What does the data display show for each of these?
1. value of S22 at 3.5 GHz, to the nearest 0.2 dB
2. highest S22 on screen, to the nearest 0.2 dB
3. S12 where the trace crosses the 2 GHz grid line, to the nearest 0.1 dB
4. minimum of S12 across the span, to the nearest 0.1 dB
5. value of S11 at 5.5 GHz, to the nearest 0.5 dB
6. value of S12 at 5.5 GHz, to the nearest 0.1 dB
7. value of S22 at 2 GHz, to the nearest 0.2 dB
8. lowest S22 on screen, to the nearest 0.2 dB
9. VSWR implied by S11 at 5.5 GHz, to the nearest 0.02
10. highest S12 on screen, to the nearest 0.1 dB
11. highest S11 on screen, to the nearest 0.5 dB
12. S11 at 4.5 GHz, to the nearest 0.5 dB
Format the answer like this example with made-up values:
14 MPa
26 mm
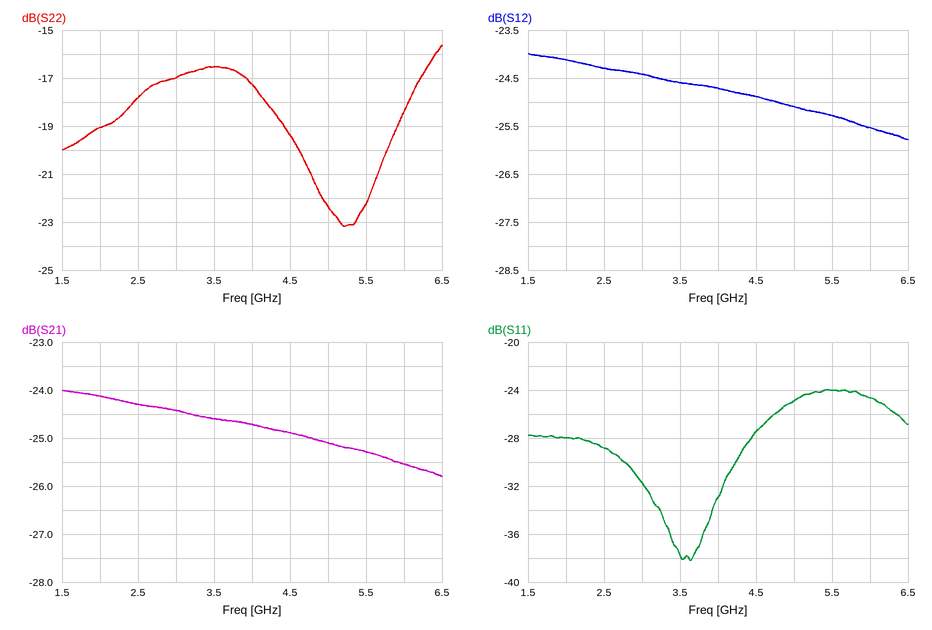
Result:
-16.6 dB
-15.6 dB
-24.1 dB
-25.8 dB
-24.0 dB
-25.3 dB
-19.0 dB
-23.2 dB
1.14
-24.0 dB
-24.0 dB
-27.5 dB
